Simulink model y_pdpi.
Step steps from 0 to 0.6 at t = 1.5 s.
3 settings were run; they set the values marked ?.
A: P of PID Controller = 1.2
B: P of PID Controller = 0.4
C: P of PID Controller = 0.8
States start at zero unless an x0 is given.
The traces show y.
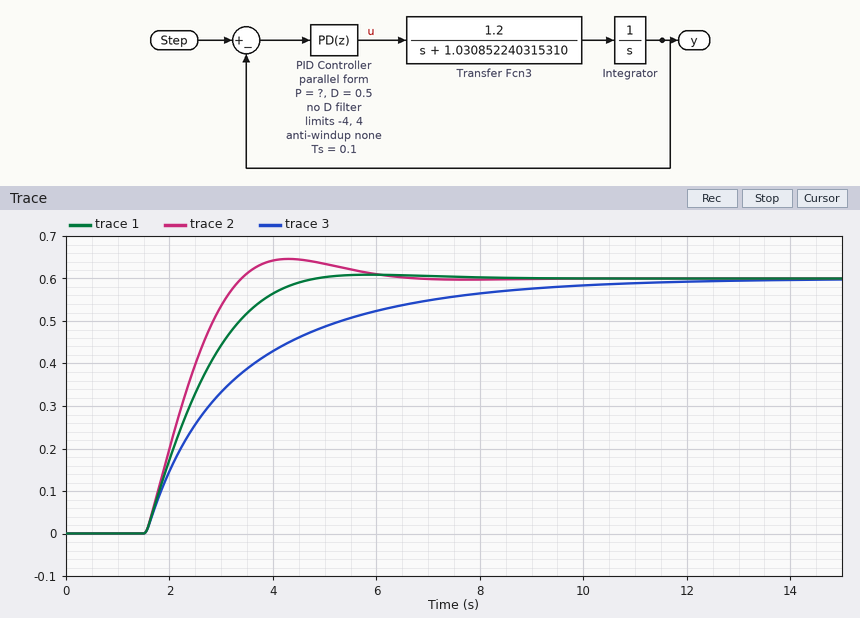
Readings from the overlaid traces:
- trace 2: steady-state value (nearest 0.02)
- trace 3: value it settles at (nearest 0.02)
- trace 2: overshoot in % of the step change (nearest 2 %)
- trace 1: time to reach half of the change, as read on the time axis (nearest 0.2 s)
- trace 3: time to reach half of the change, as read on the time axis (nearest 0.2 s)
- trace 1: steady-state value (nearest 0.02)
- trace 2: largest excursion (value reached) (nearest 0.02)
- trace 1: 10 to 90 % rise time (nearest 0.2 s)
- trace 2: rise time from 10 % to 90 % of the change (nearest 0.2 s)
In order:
0.60
0.60
8 %
2.4 s
2.8 s
0.60
0.64
2.0 s
1.4 s
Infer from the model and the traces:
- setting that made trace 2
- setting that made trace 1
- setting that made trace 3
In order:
A
C
B
